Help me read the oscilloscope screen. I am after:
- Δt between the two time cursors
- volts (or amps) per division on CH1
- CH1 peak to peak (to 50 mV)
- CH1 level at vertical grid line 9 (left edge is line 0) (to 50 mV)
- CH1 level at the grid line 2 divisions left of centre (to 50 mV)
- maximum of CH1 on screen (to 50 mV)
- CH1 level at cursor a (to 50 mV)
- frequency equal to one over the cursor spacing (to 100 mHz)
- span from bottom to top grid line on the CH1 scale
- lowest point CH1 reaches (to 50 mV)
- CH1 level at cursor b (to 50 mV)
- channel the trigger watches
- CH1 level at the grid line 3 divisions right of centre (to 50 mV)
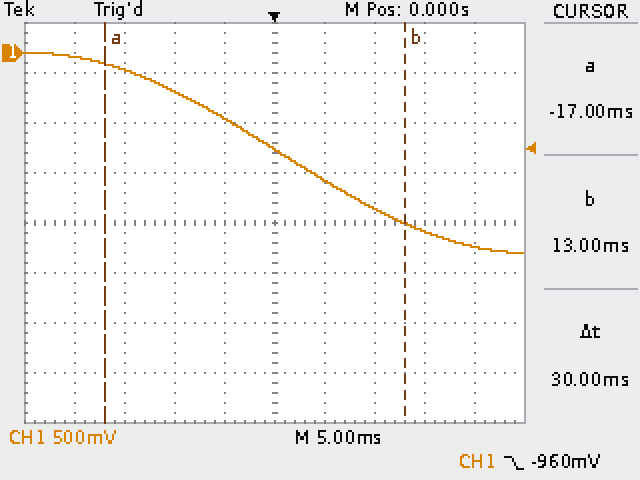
30 ms
500 mV
2.00 V
-1.95 V
-400 mV
0 mV
-100 mV
33.3 Hz
4 V
-2.00 V
-1.70 V
CH1
-1.80 V
